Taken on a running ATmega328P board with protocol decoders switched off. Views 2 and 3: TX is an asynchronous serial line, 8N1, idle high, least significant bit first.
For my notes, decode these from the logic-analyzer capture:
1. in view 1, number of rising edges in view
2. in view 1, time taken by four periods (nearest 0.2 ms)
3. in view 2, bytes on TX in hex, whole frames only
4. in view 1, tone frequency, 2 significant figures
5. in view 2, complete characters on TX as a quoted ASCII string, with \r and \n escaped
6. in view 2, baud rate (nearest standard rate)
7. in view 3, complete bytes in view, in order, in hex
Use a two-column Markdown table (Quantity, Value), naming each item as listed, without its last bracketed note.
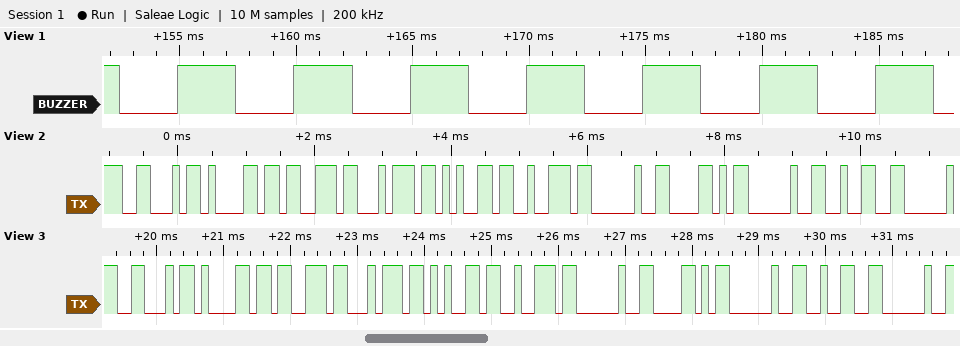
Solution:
| Quantity | Value |
|---|---|
| in view 1, number of rising edges in view | 7 |
| in view 1, time taken by four periods | 20.0 ms |
| in view 2, bytes on TX in hex, whole frames only | 0x46 0x61 0x73 0x74 0x65 0x72 0x20 0x58 0x20 0x32 |
| in view 1, tone frequency, 2 significant figures | 200 Hz |
| in view 2, complete characters on TX as a quoted ASCII string, with \r and \n escaped | "Faster X 2" |
| in view 2, baud rate | 9600 baud |
| in view 3, complete bytes in view, in order, in hex | 46 61 73 74 65 72 20 58 20 32 20 |
